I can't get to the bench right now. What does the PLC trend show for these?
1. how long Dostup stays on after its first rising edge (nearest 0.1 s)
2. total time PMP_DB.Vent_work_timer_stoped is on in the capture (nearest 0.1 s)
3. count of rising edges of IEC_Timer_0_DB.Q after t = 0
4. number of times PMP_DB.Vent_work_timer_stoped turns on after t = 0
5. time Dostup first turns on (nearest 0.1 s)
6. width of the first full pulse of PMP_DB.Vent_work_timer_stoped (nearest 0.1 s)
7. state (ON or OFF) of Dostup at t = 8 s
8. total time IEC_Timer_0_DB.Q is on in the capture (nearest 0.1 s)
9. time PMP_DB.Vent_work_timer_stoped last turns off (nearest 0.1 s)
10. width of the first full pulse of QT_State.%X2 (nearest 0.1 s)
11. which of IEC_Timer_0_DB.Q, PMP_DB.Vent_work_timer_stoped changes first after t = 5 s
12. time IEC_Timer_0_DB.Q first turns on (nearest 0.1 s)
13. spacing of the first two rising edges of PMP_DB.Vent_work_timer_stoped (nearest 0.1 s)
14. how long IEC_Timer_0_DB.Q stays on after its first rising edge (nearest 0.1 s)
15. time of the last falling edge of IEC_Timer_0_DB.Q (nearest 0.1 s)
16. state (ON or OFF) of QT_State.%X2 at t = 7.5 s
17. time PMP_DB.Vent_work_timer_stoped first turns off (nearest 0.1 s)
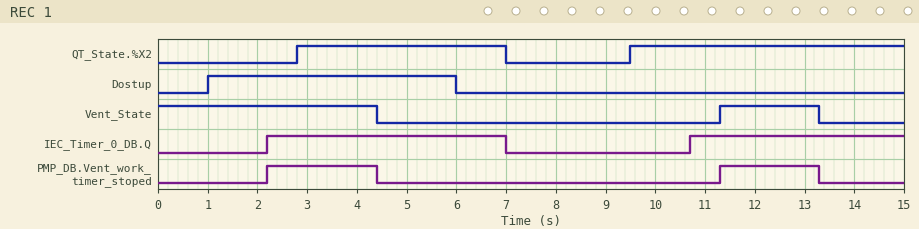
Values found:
5.0 s
4.2 s
2
2
1.0 s
2.2 s
OFF
9.1 s
13.3 s
4.2 s
IEC_Timer_0_DB.Q
2.2 s
9.1 s
4.8 s
7.0 s
OFF
4.4 s
